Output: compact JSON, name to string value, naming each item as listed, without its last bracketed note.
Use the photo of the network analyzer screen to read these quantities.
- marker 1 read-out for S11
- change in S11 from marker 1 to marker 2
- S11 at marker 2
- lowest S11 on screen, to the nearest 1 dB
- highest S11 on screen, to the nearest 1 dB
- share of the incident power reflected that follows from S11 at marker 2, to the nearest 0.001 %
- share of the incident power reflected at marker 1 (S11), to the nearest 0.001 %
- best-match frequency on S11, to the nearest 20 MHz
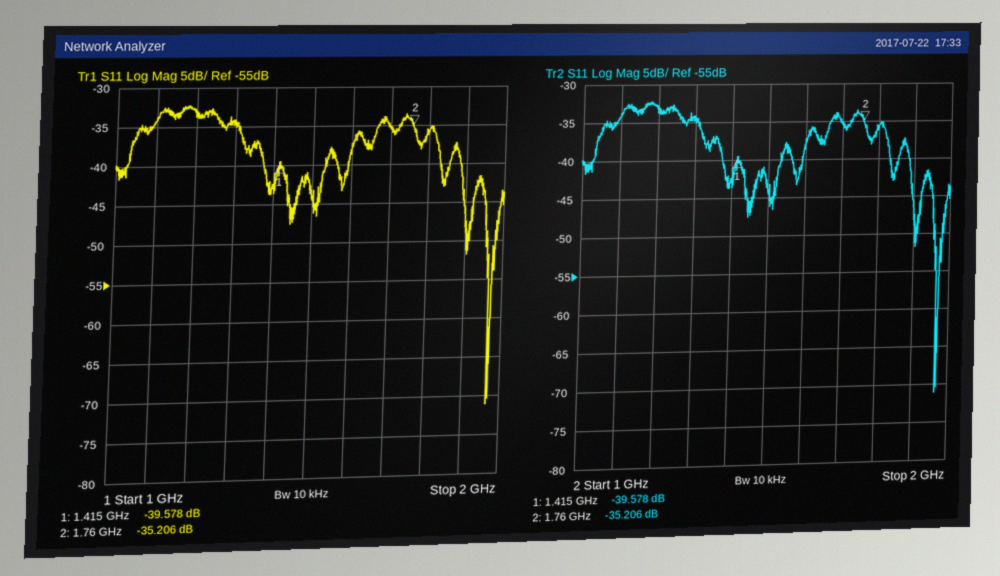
{"marker 1 read-out for S11": "-39.578 dB", "change in S11 from marker 1 to marker 2": "4.372 dB", "S11 at marker 2": "-35.206 dB", "lowest S11 on screen, to the nearest 1 dB": "-71 dB", "highest S11 on screen, to the nearest 1 dB": "-32 dB", "share of the incident power reflected that follows from S11 at marker 2, to the nearest 0.001 %": "0.030 %", "share of the incident power reflected at marker 1 (S11), to the nearest 0.001 %": "0.011 %", "best-match frequency on S11, to the nearest 20 MHz": "1.96 GHz"}
